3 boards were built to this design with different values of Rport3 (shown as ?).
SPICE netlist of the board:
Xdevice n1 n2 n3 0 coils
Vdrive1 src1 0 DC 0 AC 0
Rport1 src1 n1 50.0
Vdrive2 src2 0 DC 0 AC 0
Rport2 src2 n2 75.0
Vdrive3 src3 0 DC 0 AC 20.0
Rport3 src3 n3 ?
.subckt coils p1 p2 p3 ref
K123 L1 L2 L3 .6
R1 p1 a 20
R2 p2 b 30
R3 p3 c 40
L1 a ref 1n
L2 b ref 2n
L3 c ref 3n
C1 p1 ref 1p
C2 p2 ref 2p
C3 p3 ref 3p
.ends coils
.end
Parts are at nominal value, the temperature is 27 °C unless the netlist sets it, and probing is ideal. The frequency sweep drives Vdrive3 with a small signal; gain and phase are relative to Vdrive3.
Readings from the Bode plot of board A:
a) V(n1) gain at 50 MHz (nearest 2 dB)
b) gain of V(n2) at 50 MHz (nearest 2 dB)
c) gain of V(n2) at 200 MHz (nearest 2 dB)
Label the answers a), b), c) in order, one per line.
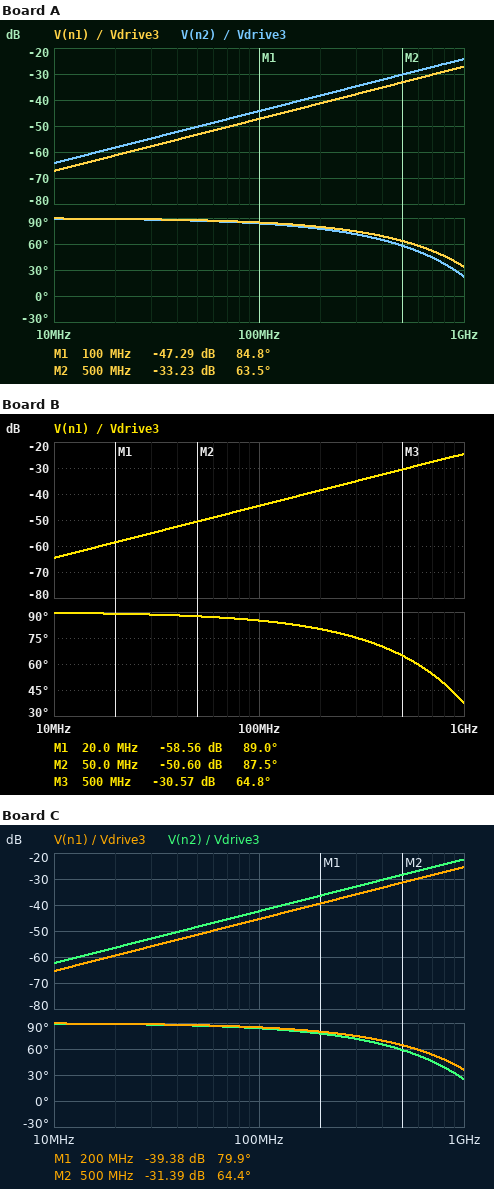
a) -54 dB
b) -50 dB
c) -38 dB
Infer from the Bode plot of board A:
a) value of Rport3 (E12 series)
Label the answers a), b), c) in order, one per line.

a) 68 Ω
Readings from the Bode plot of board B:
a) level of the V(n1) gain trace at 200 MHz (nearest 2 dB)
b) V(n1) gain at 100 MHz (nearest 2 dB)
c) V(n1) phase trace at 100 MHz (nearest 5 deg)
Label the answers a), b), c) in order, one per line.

a) -38 dB
b) -44 dB
c) 85 deg
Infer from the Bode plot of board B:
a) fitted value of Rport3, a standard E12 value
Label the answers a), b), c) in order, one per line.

a) 39 Ω
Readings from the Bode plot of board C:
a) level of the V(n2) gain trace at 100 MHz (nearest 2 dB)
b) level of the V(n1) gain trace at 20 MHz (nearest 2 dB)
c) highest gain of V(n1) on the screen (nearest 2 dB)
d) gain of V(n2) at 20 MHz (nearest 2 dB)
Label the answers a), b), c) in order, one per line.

a) -42 dB
b) -60 dB
c) -26 dB
d) -56 dB
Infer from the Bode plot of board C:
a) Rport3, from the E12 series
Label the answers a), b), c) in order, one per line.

a) 47 Ω
